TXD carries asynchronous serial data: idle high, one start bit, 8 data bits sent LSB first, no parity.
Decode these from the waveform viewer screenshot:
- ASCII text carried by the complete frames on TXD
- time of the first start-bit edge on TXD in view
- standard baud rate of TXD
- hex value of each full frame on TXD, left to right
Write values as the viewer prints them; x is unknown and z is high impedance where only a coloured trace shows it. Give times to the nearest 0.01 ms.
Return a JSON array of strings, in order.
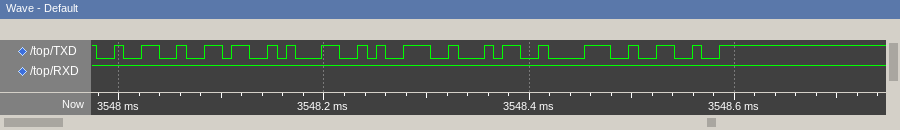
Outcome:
["\"261948&\"", "3547.98 ms", "115200 baud", "32, 36, 31, 39, 34, 38, 26"]
